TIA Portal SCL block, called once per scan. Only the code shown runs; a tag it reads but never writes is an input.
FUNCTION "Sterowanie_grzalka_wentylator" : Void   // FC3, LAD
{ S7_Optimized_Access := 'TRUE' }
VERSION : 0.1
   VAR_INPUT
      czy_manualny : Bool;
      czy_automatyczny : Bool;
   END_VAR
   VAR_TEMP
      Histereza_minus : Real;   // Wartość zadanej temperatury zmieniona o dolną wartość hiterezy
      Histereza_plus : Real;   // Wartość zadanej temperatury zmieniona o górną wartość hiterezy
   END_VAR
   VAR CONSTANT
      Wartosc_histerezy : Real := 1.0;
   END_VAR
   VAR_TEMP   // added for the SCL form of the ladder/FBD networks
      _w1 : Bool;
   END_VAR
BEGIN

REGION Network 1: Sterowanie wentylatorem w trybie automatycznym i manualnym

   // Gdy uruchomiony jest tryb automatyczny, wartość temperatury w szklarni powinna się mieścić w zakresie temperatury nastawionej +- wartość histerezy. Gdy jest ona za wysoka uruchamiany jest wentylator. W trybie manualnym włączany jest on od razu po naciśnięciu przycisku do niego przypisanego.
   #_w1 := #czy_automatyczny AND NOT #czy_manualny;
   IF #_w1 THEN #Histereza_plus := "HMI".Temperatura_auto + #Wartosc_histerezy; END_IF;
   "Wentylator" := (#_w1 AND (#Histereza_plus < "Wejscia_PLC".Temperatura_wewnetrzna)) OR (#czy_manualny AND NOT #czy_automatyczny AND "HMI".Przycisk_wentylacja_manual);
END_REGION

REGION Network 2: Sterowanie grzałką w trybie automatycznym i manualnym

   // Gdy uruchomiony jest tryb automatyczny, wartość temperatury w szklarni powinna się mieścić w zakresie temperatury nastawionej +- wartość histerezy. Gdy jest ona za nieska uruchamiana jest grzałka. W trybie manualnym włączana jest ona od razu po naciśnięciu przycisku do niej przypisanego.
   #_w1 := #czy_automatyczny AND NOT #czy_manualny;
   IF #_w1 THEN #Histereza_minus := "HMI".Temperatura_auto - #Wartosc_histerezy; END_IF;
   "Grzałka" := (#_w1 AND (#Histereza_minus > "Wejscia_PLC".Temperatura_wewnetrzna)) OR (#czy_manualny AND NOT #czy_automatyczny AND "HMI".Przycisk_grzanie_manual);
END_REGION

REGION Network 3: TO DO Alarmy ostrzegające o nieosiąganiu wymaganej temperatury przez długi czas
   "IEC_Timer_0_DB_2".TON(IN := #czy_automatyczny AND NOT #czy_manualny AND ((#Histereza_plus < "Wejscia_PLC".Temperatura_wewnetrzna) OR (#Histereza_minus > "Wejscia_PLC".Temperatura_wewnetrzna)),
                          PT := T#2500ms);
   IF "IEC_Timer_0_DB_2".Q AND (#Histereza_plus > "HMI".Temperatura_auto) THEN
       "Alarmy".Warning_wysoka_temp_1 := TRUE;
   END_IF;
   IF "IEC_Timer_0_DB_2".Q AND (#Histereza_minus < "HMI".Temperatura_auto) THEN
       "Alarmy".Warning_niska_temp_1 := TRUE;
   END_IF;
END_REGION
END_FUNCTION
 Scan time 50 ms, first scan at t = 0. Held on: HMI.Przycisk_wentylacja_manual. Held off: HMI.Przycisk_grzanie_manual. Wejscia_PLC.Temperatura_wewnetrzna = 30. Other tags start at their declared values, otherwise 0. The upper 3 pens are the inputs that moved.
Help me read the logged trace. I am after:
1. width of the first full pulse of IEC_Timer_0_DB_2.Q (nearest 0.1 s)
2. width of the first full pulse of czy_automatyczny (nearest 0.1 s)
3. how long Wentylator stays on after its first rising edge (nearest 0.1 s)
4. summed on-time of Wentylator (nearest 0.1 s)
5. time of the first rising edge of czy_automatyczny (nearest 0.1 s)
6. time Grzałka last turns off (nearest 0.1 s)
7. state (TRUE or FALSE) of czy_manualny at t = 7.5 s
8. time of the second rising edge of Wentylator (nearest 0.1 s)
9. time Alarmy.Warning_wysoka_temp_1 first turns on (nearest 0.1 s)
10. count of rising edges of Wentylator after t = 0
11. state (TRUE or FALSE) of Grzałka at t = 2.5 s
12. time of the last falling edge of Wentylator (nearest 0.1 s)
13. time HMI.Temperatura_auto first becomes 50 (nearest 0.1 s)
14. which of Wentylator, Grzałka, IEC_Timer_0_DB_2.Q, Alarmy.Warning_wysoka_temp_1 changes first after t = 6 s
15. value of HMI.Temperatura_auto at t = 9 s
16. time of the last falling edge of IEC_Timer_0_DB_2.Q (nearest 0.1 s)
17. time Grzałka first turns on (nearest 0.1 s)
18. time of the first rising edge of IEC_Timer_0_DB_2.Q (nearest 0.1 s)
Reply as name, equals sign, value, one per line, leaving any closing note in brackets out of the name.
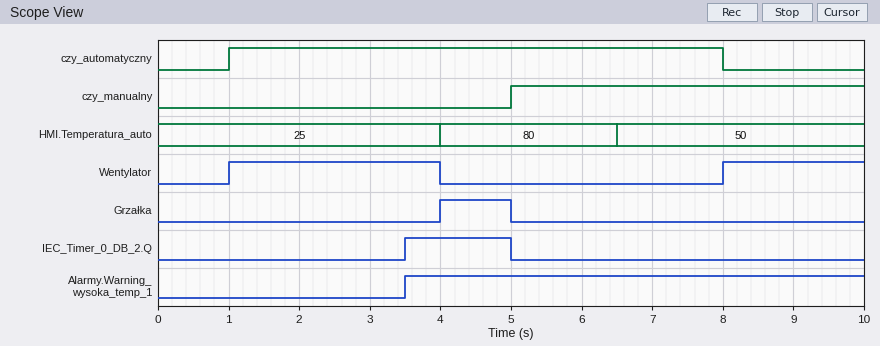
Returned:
width of the first full pulse of IEC_Timer_0_DB_2.Q = 1.5 s
width of the first full pulse of czy_automatyczny = 7.0 s
how long Wentylator stays on after its first rising edge = 3.0 s
summed on-time of Wentylator = 5.0 s
time of the first rising edge of czy_automatyczny = 1.0 s
time Grzałka last turns off = 5.0 s
state (TRUE or FALSE) of czy_manualny at t = 7.5 s = TRUE
time of the second rising edge of Wentylator = 8.0 s
time Alarmy.Warning_wysoka_temp_1 first turns on = 3.5 s
count of rising edges of Wentylator after t = 0 = 2
state (TRUE or FALSE) of Grzałka at t = 2.5 s = FALSE
time of the last falling edge of Wentylator = 4.0 s
time HMI.Temperatura_auto first becomes 50 = 6.5 s
which of Wentylator, Grzałka, IEC_Timer_0_DB_2.Q, Alarmy.Warning_wysoka_temp_1 changes first after t = 6 s = Wentylator
value of HMI.Temperatura_auto at t = 9 s = 50
time of the last falling edge of IEC_Timer_0_DB_2.Q = 5.0 s
time Grzałka first turns on = 4.0 s
time of the first rising edge of IEC_Timer_0_DB_2.Q = 3.5 s
